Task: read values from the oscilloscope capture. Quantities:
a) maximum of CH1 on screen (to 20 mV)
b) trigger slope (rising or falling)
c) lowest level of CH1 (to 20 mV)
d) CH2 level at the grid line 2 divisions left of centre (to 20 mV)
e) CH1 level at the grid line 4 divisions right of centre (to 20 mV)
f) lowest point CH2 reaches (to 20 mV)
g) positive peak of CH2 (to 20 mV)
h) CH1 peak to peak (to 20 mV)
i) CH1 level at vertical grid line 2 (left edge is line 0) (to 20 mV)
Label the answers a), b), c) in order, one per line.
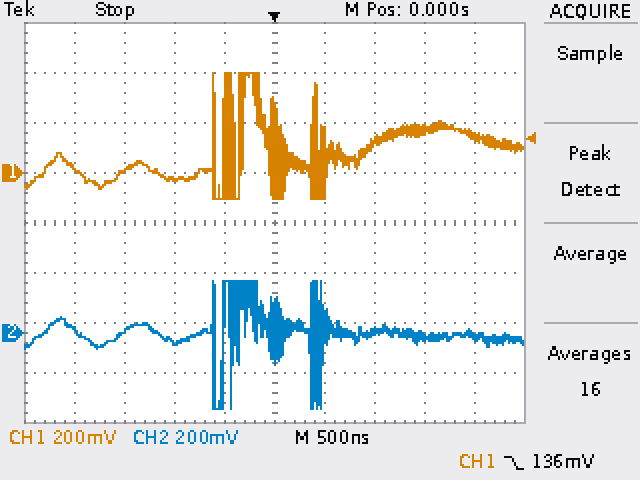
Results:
a) 400 mV
b) falling
c) -100 mV
d) -40 mV
e) 140 mV
f) -300 mV
g) 200 mV
h) 500 mV
i) 20 mV
